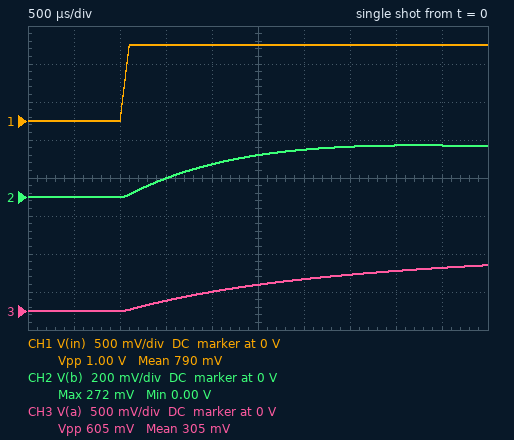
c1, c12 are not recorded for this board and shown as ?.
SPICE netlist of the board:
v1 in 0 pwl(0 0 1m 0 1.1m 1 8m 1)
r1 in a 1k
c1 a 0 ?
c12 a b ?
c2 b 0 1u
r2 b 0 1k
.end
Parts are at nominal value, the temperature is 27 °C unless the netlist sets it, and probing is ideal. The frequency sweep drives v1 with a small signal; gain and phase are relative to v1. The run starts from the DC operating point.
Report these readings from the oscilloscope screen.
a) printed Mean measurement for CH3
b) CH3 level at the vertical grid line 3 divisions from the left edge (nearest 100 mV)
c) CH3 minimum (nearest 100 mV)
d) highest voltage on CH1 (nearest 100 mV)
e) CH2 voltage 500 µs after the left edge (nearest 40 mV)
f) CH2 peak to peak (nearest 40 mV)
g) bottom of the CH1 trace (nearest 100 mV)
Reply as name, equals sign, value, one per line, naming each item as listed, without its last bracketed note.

printed Mean measurement for CH3 = 305 mV
CH3 level at the vertical grid line 3 divisions from the left edge = 100 mV
CH3 minimum = 0 V
highest voltage on CH1 = 1.0 V
CH2 voltage 500 µs after the left edge = 0 V
CH2 peak to peak = 280 mV
bottom of the CH1 trace = 0 V
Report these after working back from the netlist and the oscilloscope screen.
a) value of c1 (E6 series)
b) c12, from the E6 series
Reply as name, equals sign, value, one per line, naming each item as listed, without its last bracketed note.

value of c1 = 2.2 µF
c12, from the E6 series = 3.3 µF
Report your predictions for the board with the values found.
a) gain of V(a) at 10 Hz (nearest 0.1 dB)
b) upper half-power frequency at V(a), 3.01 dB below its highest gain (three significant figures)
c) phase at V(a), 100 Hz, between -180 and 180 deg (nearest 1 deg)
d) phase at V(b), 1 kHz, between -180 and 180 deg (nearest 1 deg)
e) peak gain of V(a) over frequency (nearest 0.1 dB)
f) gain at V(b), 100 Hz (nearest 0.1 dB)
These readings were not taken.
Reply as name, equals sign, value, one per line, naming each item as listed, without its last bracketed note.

gain of V(a) at 10 Hz = -0.8 dB
upper half-power frequency at V(a), 3.01 dB below its highest gain = 25.9 Hz
phase at V(a), 100 Hz, between -180 and 180 deg = -54 deg
phase at V(b), 1 kHz, between -180 and 180 deg = -83 deg
peak gain of V(a) over frequency = 0 dB
gain at V(b), 100 Hz = -11.0 dB
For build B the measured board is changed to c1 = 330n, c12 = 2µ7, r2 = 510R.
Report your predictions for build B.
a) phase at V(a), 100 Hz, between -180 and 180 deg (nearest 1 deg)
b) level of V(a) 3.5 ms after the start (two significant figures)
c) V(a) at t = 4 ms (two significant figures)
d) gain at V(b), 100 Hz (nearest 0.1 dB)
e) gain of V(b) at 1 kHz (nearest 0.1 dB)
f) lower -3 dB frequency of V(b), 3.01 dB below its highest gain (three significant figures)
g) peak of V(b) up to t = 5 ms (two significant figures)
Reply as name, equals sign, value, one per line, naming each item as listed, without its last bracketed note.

phase at V(a), 100 Hz, between -180 and 180 deg = -36 deg
level of V(a) 3.5 ms after the start = 630 mV
V(a) at t = 4 ms = 670 mV
gain at V(b), 100 Hz = -11.1 dB
gain of V(b) at 1 kHz = -19.7 dB
lower -3 dB frequency of V(b), 3.01 dB below its highest gain = 30.1 Hz
peak of V(b) up to t = 5 ms = 240 mV
